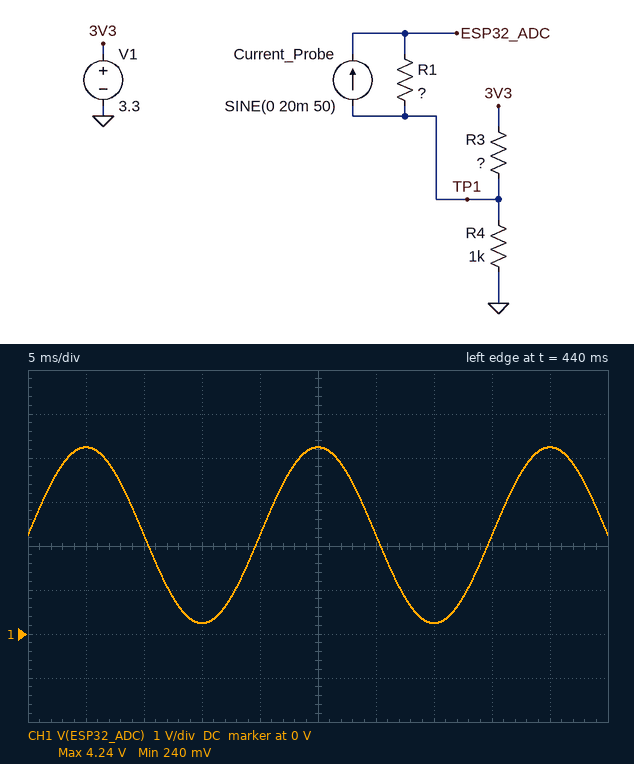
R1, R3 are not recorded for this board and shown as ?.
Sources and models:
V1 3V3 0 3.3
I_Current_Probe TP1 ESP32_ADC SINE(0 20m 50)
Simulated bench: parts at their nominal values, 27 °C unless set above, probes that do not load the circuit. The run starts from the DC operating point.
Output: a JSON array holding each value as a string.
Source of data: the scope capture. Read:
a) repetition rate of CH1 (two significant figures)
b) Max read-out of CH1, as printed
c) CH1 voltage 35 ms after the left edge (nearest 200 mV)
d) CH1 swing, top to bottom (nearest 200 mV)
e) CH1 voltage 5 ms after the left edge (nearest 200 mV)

["50 Hz", "4.24 V", "200 mV", "4.0 V", "4.2 V"]
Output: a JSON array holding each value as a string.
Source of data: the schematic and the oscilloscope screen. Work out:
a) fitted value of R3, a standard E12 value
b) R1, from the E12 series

["470 Ω", "100 Ω"]
